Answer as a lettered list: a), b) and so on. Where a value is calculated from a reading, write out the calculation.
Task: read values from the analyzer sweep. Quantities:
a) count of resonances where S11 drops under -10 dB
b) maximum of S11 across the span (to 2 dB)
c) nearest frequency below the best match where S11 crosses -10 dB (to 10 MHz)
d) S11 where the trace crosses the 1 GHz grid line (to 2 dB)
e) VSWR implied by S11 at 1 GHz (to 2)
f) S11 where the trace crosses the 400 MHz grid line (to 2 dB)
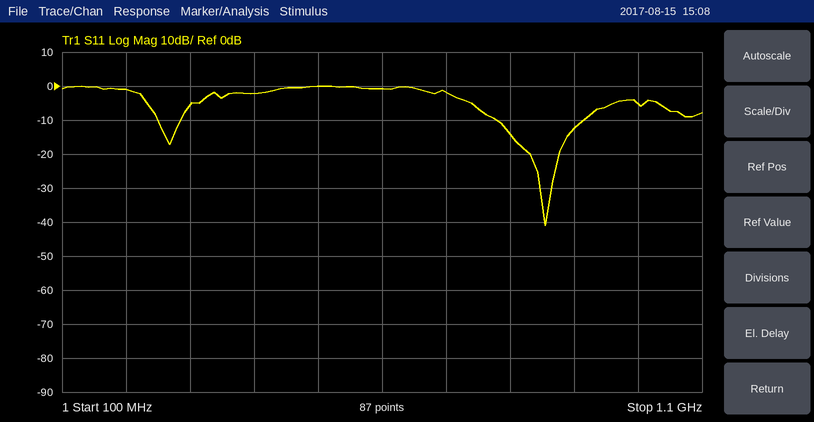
a) 2
b) 0 dB
c) 780 MHz
d) -6 dB
e) |Γ| = 10^(-6/20) = 0.5012; VSWR = (1 + 0.5012)/(1 − 0.5012) ≈ 3.01, so 4 to the nearest 2
f) -2 dB
